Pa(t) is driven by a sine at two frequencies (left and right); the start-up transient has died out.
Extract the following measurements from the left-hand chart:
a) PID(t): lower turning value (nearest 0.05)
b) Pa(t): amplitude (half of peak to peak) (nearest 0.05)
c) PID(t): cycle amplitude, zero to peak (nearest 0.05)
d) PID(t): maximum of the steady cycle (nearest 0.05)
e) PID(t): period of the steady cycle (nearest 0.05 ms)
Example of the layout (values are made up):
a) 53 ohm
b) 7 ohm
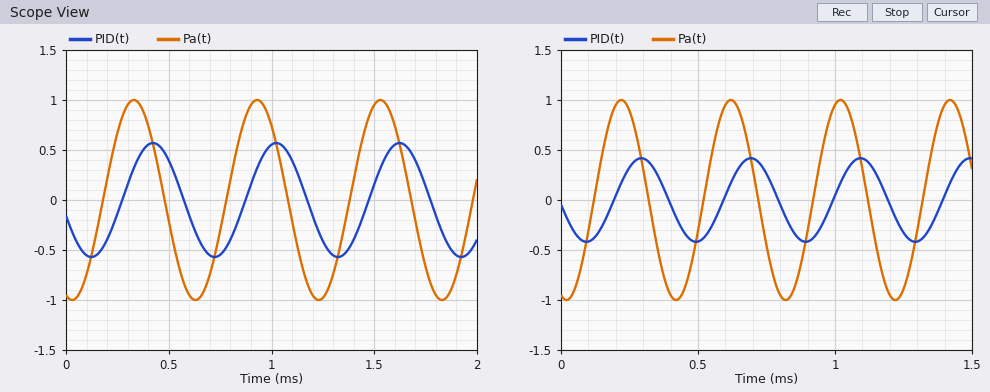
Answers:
a) -0.55
b) 1.00
c) 0.55
d) 0.55
e) 0.60 ms
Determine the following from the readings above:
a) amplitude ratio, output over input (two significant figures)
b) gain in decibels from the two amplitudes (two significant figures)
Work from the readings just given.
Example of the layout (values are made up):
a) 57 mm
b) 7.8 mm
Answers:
a) 0.55
b) -5.2 dB
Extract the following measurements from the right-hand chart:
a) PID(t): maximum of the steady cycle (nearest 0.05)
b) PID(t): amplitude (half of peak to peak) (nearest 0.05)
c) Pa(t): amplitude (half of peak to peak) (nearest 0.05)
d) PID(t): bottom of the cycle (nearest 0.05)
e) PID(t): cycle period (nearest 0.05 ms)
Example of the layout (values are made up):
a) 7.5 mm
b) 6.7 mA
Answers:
a) 0.40
b) 0.40
c) 1.00
d) -0.40
e) 0.40 ms
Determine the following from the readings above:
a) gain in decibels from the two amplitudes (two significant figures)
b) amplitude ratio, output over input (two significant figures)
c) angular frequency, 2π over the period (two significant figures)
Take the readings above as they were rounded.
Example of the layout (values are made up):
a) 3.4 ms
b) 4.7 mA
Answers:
a) -8.0 dB
b) 0.40
c) 16 rad/ms
